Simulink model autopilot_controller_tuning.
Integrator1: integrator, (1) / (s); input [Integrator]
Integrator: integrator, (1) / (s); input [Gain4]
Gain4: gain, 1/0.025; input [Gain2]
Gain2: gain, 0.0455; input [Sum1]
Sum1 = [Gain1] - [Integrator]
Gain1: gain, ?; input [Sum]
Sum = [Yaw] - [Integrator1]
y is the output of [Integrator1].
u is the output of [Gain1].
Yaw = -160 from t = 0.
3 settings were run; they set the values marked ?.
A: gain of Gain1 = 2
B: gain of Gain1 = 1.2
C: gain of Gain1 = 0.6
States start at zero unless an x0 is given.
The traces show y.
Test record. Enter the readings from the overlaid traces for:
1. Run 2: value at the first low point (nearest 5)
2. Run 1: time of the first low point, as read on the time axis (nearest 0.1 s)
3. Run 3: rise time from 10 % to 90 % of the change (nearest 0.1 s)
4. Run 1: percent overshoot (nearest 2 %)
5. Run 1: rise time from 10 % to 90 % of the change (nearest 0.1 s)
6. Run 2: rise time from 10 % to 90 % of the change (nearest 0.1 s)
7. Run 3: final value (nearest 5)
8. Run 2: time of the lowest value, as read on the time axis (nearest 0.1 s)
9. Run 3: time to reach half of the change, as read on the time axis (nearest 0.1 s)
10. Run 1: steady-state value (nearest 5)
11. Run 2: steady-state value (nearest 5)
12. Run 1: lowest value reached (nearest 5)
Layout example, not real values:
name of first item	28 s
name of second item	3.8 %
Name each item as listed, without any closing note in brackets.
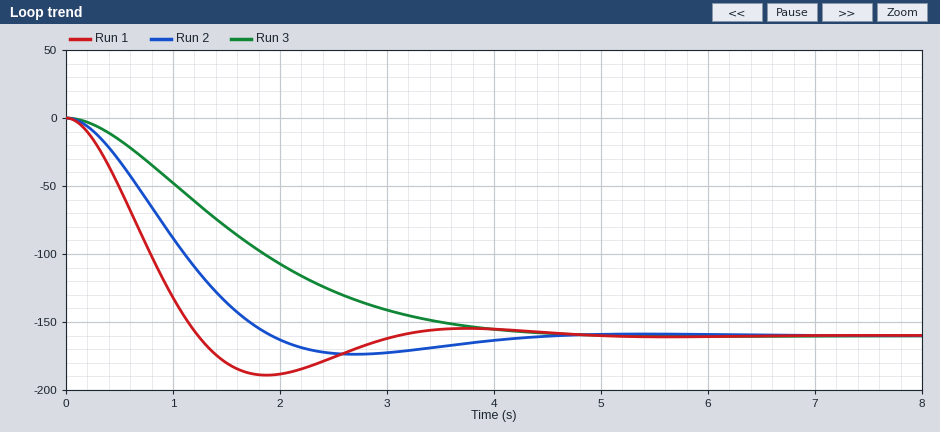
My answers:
Run 2: value at the first low point	-175
Run 1: time of the first low point, as read on the time axis	1.9 s
Run 3: rise time from 10 % to 90 % of the change	2.6 s
Run 1: percent overshoot	18 %
Run 1: rise time from 10 % to 90 % of the change	0.8 s
Run 2: rise time from 10 % to 90 % of the change	1.3 s
Run 3: final value	-160
Run 2: time of the lowest value, as read on the time axis	2.7 s
Run 3: time to reach half of the change, as read on the time axis	1.5 s
Run 1: steady-state value	-160
Run 2: steady-state value	-160
Run 1: lowest value reached	-190
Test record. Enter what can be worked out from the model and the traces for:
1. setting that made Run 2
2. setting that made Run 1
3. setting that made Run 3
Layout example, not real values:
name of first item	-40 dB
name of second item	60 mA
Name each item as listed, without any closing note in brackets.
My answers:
setting that made Run 2	B
setting that made Run 1	A
setting that made Run 3	C
